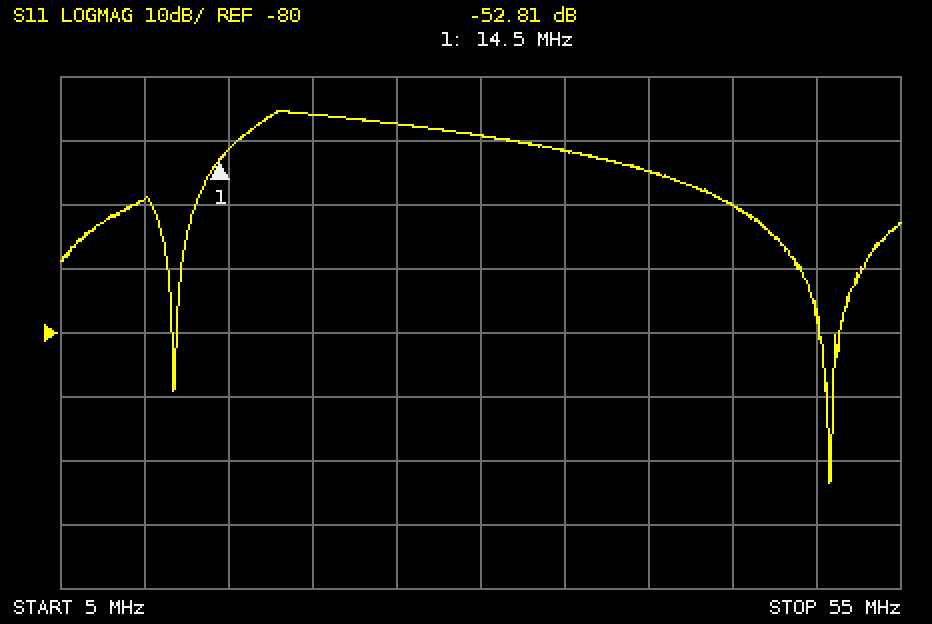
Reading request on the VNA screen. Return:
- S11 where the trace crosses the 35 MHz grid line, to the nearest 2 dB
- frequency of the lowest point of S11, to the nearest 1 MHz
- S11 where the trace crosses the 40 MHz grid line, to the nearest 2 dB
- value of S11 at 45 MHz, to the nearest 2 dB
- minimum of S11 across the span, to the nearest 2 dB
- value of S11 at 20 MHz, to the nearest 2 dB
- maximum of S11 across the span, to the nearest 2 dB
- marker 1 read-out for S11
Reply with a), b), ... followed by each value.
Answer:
a) -52 dB
b) 51 MHz
c) -54 dB
d) -60 dB
e) -104 dB
f) -46 dB
g) -46 dB
h) -52.81 dB
